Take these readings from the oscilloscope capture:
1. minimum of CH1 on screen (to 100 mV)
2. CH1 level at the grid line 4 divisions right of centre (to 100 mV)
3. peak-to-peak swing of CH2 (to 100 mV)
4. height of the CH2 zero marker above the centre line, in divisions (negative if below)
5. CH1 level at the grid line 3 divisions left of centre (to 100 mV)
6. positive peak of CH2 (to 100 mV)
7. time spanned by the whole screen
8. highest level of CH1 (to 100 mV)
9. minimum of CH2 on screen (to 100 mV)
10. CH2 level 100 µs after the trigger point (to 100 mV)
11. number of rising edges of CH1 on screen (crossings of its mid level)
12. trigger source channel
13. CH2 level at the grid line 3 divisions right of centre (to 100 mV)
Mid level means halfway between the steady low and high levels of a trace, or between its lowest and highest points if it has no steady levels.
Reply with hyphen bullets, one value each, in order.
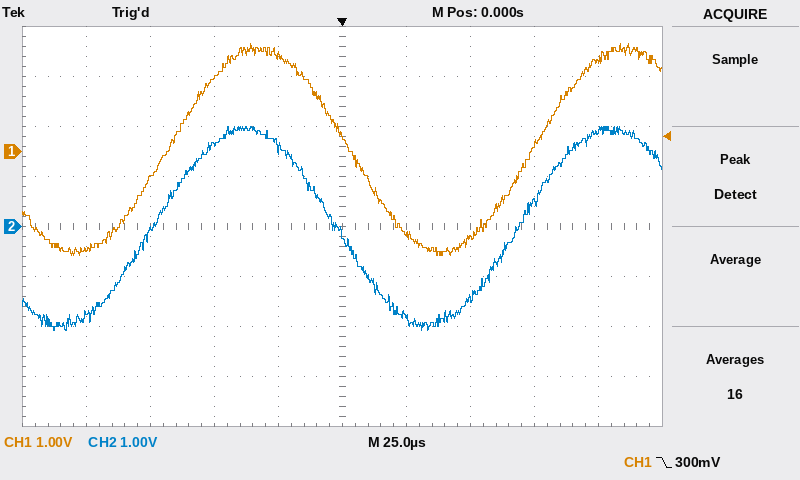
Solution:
- -2.1 V
- 1.8 V
- 4.1 V
- 0.0 div
- -600 mV
- 2.0 V
- 250 µs
- 2.2 V
- -2.1 V
- 1.9 V
- 2
- CH1
- 500 mV
